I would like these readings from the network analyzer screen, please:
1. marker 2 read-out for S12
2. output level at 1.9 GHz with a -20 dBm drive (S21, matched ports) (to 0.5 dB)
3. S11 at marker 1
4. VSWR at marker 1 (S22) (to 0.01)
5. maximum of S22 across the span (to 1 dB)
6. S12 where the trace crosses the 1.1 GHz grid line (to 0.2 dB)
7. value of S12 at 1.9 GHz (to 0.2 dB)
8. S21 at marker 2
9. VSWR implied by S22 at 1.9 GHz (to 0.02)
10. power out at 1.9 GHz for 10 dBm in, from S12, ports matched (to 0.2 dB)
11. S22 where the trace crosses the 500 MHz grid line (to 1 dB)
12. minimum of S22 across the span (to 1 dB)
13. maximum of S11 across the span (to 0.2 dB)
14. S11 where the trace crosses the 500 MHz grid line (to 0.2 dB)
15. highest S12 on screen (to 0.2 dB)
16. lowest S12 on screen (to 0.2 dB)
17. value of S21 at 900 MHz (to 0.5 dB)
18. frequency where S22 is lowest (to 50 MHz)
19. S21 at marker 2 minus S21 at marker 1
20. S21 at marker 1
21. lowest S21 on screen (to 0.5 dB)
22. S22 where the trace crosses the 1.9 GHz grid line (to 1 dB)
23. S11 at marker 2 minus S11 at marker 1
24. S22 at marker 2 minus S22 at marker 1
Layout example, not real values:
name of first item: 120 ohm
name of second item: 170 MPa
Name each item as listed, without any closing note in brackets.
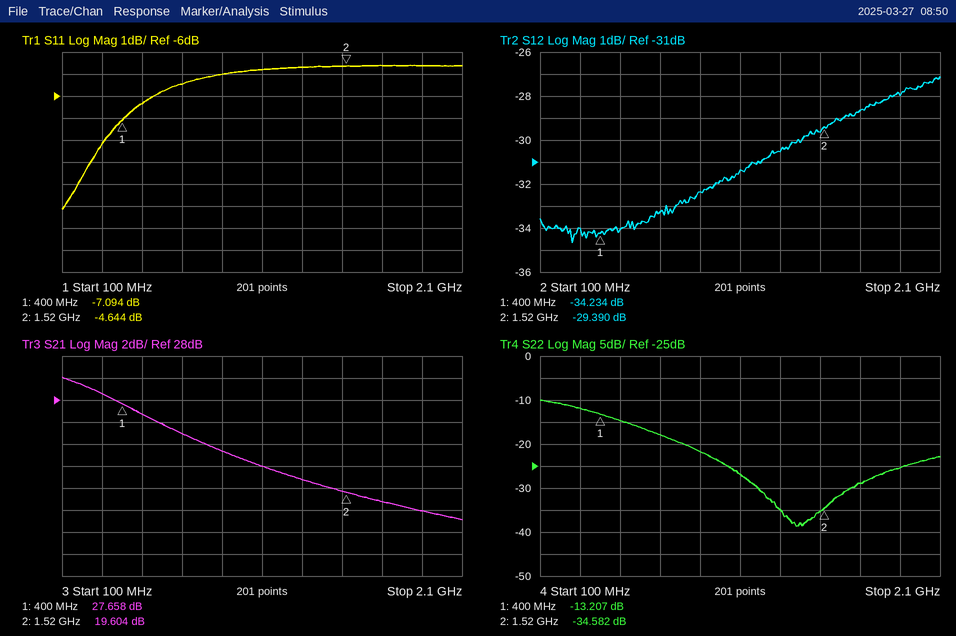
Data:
marker 2 read-out for S12: -29.390 dB
output level at 1.9 GHz with a -20 dBm drive (S21, matched ports): -2.0 dBm
S11 at marker 1: -7.094 dB
VSWR at marker 1 (S22): 1.56
maximum of S22 across the span: -10 dB
S12 where the trace crosses the 1.1 GHz grid line: -31.4 dB
value of S12 at 1.9 GHz: -28.0 dB
S21 at marker 2: 19.604 dB
VSWR implied by S22 at 1.9 GHz: 1.12
power out at 1.9 GHz for 10 dBm in, from S12, ports matched: -18.0 dBm
S22 where the trace crosses the 500 MHz grid line: -15 dB
minimum of S22 across the span: -39 dB
maximum of S11 across the span: -4.6 dB
S11 where the trace crosses the 500 MHz grid line: -6.4 dB
highest S12 on screen: -27.2 dB
lowest S12 on screen: -34.6 dB
value of S21 at 900 MHz: 23.5 dB
frequency where S22 is lowest: 1.40 GHz
S21 at marker 2 minus S21 at marker 1: -8.054 dB
S21 at marker 1: 27.658 dB
lowest S21 on screen: 17.0 dB
S22 where the trace crosses the 1.9 GHz grid line: -25 dB
S11 at marker 2 minus S11 at marker 1: 2.450 dB
S22 at marker 2 minus S22 at marker 1: -21.375 dB
